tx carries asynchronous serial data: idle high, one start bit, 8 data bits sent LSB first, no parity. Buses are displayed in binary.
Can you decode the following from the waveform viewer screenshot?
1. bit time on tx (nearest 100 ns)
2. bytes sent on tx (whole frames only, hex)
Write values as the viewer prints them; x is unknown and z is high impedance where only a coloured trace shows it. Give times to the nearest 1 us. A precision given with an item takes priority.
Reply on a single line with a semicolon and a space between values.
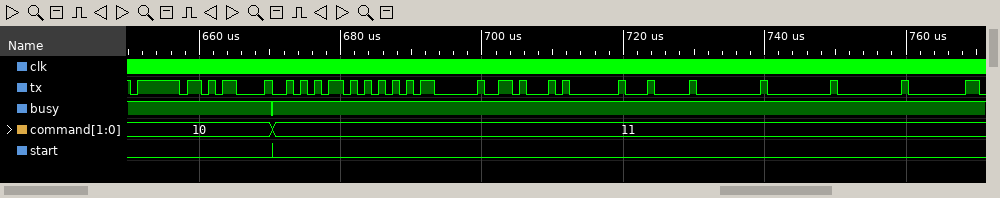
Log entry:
1000 ns; BF, 0D, AA, 55, 03, 16, 01, 04, 00, 00, 00, 80
